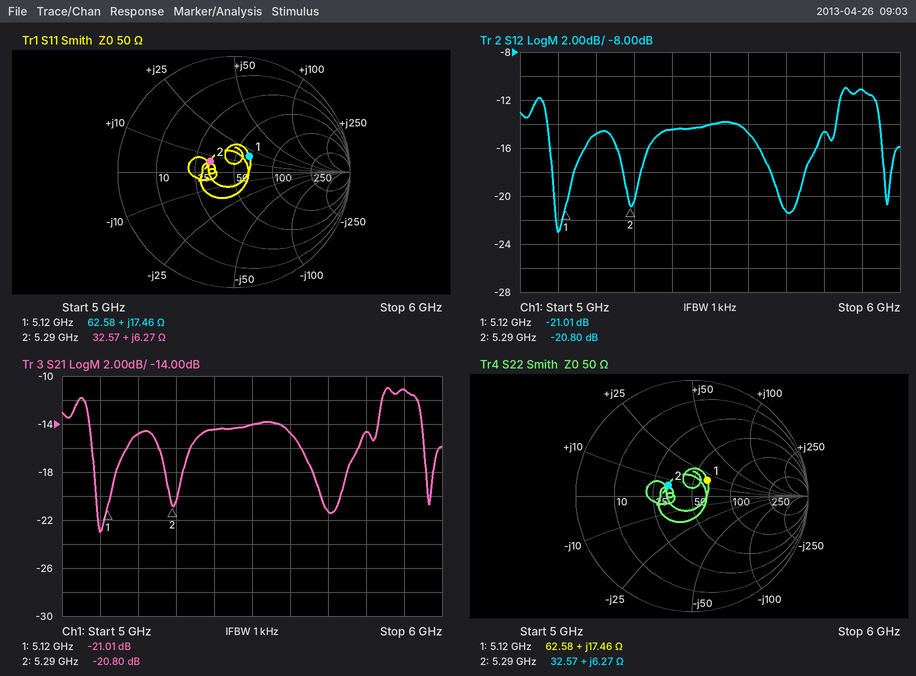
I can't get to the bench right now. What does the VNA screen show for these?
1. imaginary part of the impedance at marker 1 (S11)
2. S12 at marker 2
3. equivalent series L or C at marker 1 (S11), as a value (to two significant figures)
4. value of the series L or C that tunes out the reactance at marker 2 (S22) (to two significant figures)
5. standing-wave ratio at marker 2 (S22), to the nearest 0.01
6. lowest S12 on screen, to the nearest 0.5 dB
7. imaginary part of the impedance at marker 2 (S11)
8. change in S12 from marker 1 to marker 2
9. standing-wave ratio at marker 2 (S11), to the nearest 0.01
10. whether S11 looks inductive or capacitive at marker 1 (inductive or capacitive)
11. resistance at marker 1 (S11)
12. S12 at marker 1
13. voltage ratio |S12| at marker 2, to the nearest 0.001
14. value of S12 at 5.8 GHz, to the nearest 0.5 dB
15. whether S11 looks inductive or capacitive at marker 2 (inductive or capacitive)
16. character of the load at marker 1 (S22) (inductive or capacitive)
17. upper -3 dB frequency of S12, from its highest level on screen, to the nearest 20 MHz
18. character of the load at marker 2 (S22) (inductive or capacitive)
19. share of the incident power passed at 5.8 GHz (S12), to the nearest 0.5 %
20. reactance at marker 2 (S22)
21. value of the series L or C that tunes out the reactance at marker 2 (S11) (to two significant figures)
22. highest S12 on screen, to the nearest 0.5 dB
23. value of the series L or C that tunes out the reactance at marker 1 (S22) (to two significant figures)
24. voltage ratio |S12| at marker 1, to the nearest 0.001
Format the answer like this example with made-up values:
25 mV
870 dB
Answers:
+17.46 Ω
-20.80 dB
540 pH
4.8 pF
1.58
-23.0 dB
+6.27 Ω
0.21 dB
1.58
inductive
62.58 Ω
-21.01 dB
0.091
-14.5 dB
inductive
inductive
5.94 GHz
inductive
3.5 %
+6.27 Ω
4.8 pF
-11.0 dB
1.8 pF
0.089
